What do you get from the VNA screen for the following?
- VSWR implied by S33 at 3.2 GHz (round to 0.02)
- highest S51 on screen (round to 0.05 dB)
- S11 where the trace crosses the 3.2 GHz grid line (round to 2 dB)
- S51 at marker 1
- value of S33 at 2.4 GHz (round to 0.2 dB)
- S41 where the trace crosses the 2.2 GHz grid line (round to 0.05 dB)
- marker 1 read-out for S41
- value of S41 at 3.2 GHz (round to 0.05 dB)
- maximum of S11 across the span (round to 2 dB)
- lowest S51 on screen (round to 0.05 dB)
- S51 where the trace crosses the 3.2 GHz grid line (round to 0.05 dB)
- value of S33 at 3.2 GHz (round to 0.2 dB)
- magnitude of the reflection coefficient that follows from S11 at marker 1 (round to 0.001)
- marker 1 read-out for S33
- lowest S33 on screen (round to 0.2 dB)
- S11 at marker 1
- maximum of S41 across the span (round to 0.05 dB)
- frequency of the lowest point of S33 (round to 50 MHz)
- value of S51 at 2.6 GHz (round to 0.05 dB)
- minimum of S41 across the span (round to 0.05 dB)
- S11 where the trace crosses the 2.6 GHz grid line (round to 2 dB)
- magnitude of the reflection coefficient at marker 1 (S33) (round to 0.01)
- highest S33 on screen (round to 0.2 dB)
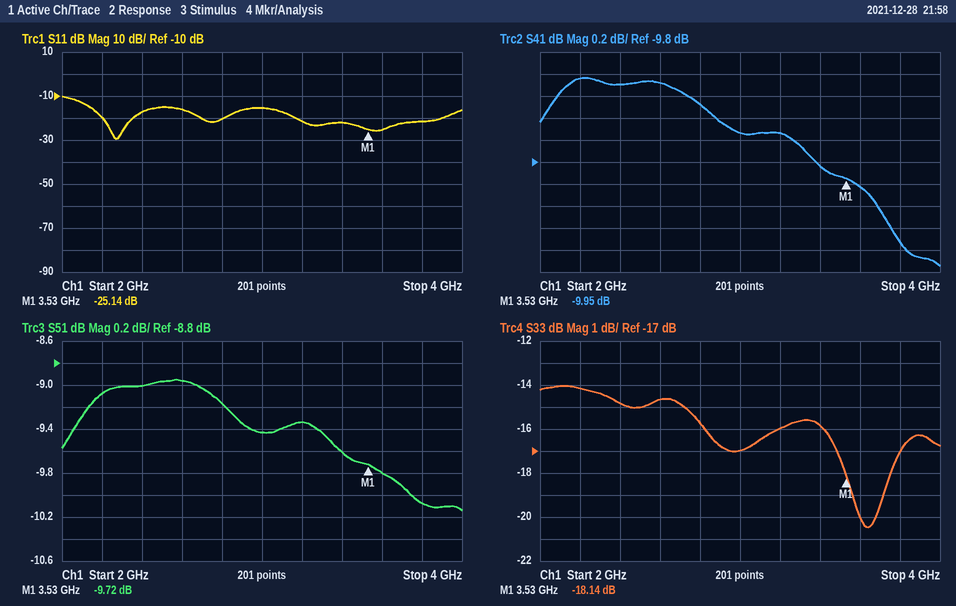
1.38
-8.95 dB
-22 dB
-9.72 dB
-14.8 dB
-9.05 dB
-9.95 dB
-9.55 dB
-10 dB
-10.15 dB
-9.35 dB
-16.0 dB
0.055
-18.14 dB
-20.4 dB
-25.14 dB
-9.05 dB
3.65 GHz
-8.95 dB
-10.75 dB
-16 dB
0.12
-14.0 dB
